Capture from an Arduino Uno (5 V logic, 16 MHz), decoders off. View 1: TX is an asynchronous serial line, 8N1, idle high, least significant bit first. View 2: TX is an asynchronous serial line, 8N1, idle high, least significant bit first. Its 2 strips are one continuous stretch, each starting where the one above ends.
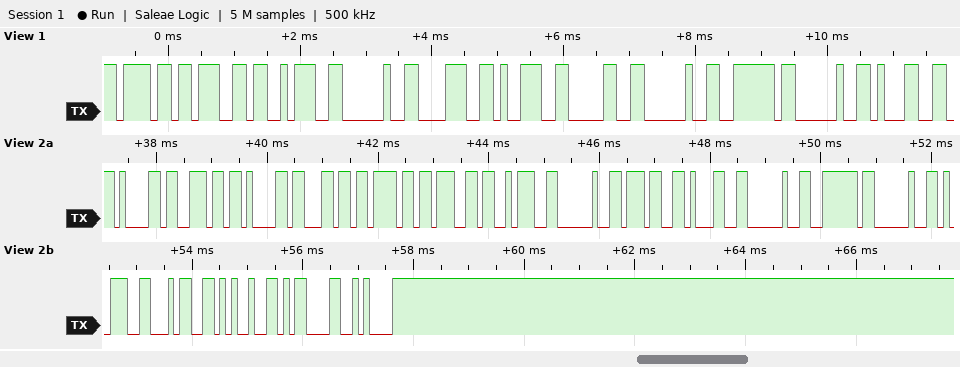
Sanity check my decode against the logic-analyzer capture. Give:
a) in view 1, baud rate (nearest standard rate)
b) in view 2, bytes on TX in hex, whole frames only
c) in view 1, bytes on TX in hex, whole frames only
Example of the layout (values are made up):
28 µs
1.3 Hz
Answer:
9600 baud
61 6E 61 6C 6F 67 3A 20 37 31 20 7E 20 39 34 25 0D 0A
6F 67 3A 20 38 39 30 20 7E 20 31
